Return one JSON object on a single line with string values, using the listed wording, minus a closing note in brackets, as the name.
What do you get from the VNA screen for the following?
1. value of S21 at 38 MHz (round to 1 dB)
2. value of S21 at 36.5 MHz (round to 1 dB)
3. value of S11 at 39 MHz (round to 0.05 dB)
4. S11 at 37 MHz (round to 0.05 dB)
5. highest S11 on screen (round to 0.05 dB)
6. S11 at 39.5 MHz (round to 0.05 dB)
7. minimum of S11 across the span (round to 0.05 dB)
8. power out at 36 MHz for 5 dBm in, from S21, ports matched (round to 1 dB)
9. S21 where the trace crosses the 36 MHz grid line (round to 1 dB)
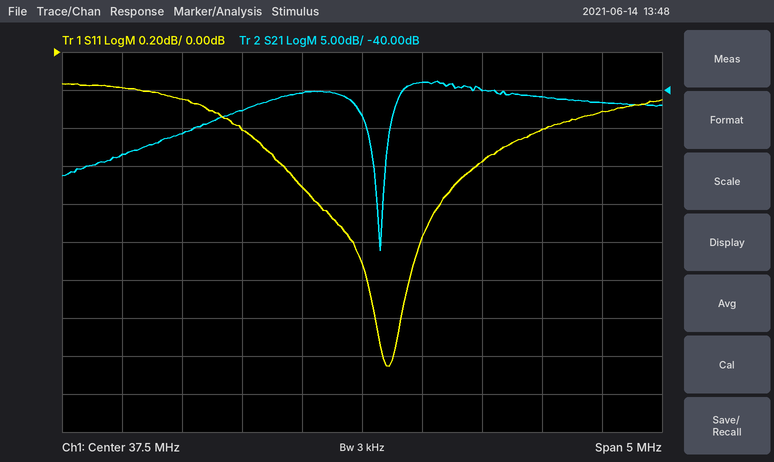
{"value of S21 at 38 MHz": "-39 dB", "value of S21 at 36.5 MHz": "-43 dB", "value of S11 at 39 MHz": "-0.40 dB", "S11 at 37 MHz": "-0.70 dB", "highest S11 on screen": "-0.15 dB", "S11 at 39.5 MHz": "-0.30 dB", "minimum of S11 across the span": "-1.65 dB", "power out at 36 MHz for 5 dBm in, from S21, ports matched": "-41 dBm", "S21 where the trace crosses the 36 MHz grid line": "-46 dB"}
